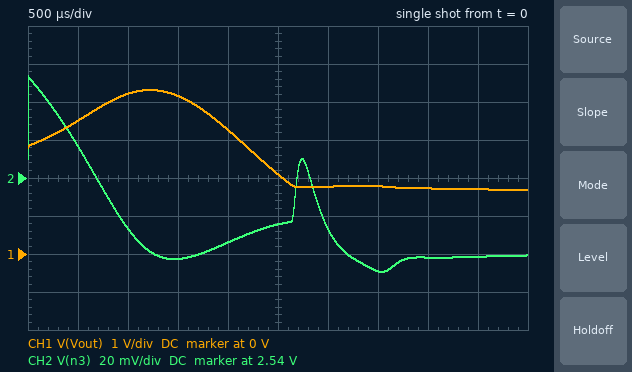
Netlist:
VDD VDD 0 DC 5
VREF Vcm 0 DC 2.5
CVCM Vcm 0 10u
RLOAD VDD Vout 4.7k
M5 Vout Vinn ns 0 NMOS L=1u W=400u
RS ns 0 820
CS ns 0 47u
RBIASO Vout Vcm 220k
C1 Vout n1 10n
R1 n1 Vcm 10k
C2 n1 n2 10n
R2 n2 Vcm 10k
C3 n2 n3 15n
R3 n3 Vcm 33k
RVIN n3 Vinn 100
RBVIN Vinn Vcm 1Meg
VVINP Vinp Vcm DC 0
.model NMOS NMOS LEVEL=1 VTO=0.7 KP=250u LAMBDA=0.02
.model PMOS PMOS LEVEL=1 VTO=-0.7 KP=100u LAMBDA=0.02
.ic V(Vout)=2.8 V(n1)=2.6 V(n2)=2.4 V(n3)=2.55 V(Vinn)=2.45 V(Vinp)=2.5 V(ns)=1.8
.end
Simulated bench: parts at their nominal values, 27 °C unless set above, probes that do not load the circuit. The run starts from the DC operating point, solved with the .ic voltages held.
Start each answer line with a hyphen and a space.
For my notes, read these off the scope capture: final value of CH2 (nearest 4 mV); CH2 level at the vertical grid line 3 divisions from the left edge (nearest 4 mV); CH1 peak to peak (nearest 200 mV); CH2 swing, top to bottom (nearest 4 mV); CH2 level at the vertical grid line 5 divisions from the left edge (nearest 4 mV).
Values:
- 2.500 V
- 2.496 V
- 2.6 V
- 104 mV
- 2.516 V
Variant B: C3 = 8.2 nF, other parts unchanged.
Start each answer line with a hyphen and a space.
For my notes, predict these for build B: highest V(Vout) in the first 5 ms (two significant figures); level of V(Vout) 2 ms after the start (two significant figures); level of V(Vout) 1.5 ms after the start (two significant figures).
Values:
- 4.9 V
- 2.5 V
- 3.9 V
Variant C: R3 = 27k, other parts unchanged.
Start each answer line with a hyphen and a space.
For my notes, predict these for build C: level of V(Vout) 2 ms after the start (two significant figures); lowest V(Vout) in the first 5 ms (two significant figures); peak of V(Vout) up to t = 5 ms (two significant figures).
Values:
- 3.0 V
- 1.7 V
- 4.6 V
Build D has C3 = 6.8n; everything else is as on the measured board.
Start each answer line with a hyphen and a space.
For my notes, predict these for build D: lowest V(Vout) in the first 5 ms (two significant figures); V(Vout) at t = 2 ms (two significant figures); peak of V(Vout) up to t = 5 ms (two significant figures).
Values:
- 1.7 V
- 2.5 V
- 4.9 V
